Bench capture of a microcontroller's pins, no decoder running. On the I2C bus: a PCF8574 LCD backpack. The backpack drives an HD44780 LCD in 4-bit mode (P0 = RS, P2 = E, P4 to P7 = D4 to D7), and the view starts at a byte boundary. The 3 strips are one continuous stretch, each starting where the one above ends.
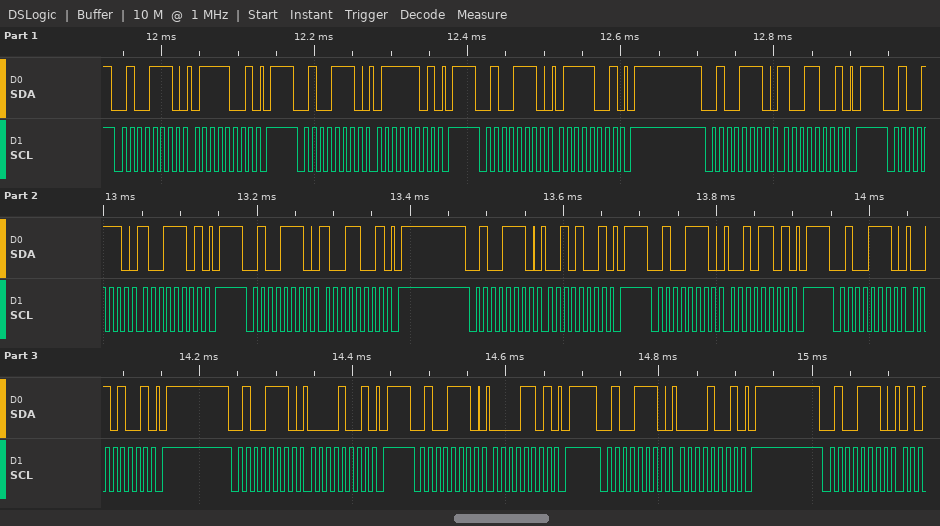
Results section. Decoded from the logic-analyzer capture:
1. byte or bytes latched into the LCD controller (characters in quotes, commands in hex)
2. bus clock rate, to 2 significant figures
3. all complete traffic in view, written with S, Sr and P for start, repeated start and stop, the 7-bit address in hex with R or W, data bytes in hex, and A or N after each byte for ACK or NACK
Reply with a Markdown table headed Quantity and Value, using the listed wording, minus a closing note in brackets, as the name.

| Quantity | Value |
|---|---|
| byte or bytes latched into the LCD controller | 'y' ' ' |
| bus clock rate, to 2 significant figures | 100 kHz |
| all complete traffic in view, written with S, Sr and P for start, repeated start and stop, the 7-bit address in hex with R or W, data bytes in hex, and A or N after each byte for ACK or NACK | S 27W A 79 A P S 27W A 7D A P S 27W A 79 A P S 27W A 99 A P S 27W A 9D A P S 27W A 99 A P S 27W A 29 A P S 27W A 2D A P S 27W A 29 A P S 27W A 09 A P S 27W A 0D A P S 27W A 09 A P S 27W A |
